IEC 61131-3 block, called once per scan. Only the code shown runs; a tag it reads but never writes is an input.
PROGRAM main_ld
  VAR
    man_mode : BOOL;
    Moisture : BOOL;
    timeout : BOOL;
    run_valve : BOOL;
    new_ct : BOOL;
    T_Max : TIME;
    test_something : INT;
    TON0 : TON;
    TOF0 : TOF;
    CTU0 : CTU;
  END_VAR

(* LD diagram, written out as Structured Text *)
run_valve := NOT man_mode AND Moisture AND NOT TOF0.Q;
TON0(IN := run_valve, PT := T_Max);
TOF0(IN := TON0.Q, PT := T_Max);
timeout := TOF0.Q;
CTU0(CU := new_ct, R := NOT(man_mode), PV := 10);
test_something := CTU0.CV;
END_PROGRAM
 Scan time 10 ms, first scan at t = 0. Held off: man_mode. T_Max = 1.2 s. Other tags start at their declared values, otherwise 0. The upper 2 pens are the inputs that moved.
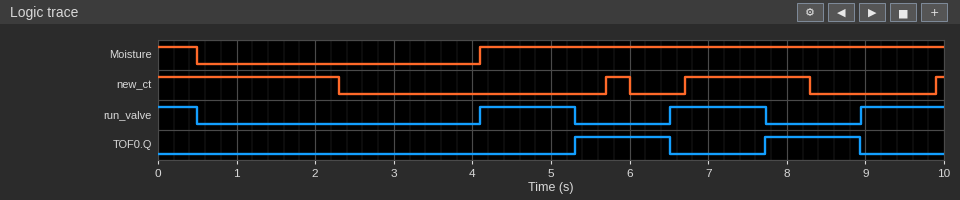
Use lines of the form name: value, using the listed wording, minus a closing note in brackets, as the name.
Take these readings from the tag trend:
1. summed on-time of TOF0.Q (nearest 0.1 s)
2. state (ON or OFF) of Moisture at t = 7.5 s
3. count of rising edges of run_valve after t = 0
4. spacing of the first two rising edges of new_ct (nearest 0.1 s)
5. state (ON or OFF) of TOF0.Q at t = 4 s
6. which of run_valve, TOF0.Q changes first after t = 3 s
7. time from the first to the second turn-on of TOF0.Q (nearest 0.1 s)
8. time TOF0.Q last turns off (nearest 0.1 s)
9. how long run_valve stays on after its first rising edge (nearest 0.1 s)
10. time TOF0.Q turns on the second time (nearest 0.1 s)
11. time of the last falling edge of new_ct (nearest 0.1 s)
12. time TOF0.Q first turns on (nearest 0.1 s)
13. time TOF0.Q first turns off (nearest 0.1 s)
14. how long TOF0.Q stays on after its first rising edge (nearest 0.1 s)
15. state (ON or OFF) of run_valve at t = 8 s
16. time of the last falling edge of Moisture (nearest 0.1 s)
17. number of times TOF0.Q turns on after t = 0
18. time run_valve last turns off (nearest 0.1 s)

summed on-time of TOF0.Q: 2.4 s
state (ON or OFF) of Moisture at t = 7.5 s: ON
count of rising edges of run_valve after t = 0: 3
spacing of the first two rising edges of new_ct: 1.0 s
state (ON or OFF) of TOF0.Q at t = 4 s: OFF
which of run_valve, TOF0.Q changes first after t = 3 s: run_valve
time from the first to the second turn-on of TOF0.Q: 2.4 s
time TOF0.Q last turns off: 8.9 s
how long run_valve stays on after its first rising edge: 1.2 s
time TOF0.Q turns on the second time: 7.7 s
time of the last falling edge of new_ct: 8.3 s
time TOF0.Q first turns on: 5.3 s
time TOF0.Q first turns off: 6.5 s
how long TOF0.Q stays on after its first rising edge: 1.2 s
state (ON or OFF) of run_valve at t = 8 s: OFF
time of the last falling edge of Moisture: 0.5 s
number of times TOF0.Q turns on after t = 0: 2
time run_valve last turns off: 7.7 s
